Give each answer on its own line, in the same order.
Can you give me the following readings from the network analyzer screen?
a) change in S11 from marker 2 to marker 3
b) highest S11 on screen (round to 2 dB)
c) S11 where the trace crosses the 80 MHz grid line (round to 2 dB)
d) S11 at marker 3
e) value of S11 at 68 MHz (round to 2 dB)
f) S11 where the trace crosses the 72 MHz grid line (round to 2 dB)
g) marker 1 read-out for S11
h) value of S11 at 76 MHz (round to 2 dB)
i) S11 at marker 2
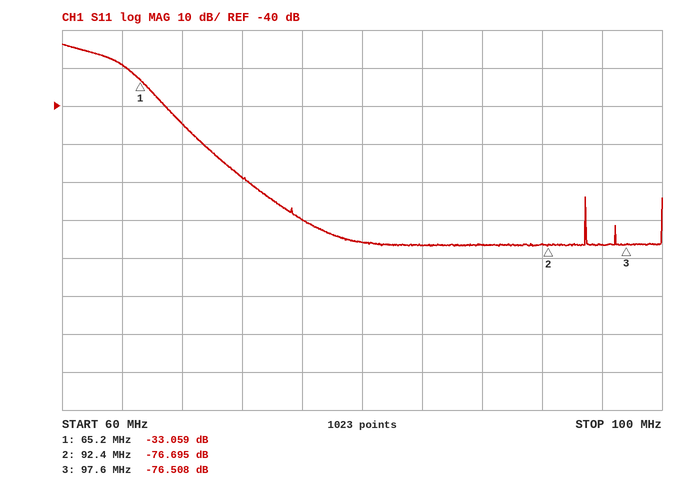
0.187 dB
-24 dB
-76 dB
-76.508 dB
-44 dB
-58 dB
-33.059 dB
-70 dB
-76.695 dB
